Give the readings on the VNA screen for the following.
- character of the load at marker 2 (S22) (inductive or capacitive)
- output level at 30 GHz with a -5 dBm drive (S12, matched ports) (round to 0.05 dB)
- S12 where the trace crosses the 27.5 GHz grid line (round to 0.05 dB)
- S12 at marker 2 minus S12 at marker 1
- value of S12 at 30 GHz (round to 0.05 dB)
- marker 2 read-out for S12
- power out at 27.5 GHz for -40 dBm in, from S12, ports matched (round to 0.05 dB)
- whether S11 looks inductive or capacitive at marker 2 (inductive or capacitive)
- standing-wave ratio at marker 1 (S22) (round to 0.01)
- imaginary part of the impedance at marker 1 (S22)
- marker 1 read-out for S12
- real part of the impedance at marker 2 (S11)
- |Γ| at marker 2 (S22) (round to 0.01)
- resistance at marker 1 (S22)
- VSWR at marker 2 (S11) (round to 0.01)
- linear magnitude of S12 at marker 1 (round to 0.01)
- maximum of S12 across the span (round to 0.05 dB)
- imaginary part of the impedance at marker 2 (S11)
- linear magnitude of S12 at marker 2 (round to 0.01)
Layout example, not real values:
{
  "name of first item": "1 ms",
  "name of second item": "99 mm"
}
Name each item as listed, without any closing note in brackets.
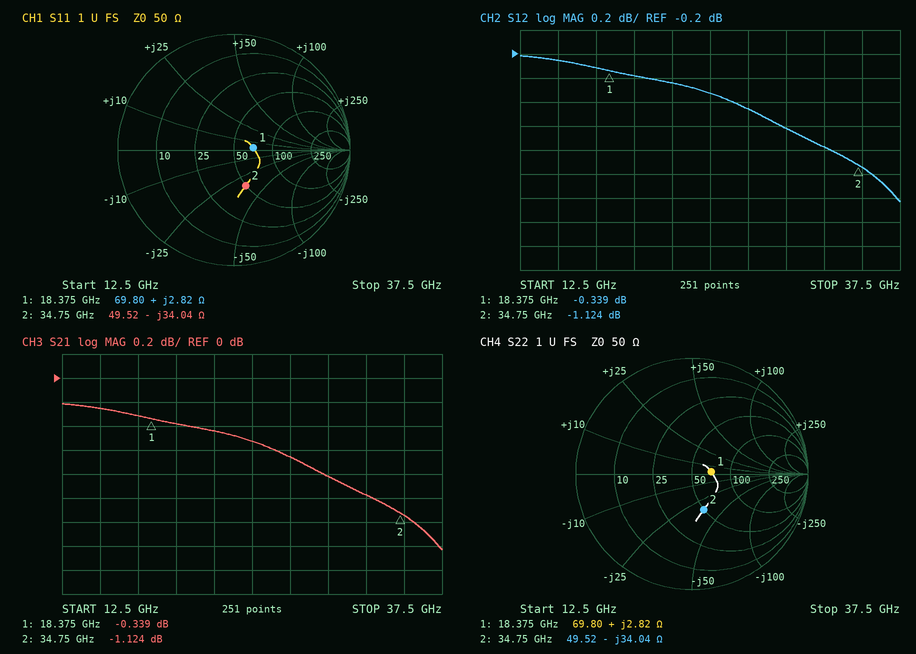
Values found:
{
  "character of the load at marker 2 (S22)": "capacitive",
  "output level at 30 GHz with a -5 dBm drive (S12, matched ports)": "-5.80 dBm",
  "S12 where the trace crosses the 27.5 GHz grid line": "-0.65 dB",
  "S12 at marker 2 minus S12 at marker 1": "-0.785 dB",
  "value of S12 at 30 GHz": "-0.80 dB",
  "marker 2 read-out for S12": "-1.124 dB",
  "power out at 27.5 GHz for -40 dBm in, from S12, ports matched": "-40.65 dBm",
  "whether S11 looks inductive or capacitive at marker 2": "capacitive",
  "standing-wave ratio at marker 1 (S22)": "1.40",
  "imaginary part of the impedance at marker 1": "+2.82 Ω",
  "marker 1 read-out for S12": "-0.339 dB",
  "real part of the impedance at marker 2": "49.52 Ω",
  "|Γ| at marker 2 (S22)": "0.32",
  "resistance at marker 1": "69.80 Ω",
  "VSWR at marker 2 (S11)": "1.96",
  "linear magnitude of S12 at marker 1": "0.96",
  "maximum of S12 across the span": "-0.20 dB",
  "imaginary part of the impedance at marker 2": "-34.04 Ω",
  "linear magnitude of S12 at marker 2": "0.88"
}
